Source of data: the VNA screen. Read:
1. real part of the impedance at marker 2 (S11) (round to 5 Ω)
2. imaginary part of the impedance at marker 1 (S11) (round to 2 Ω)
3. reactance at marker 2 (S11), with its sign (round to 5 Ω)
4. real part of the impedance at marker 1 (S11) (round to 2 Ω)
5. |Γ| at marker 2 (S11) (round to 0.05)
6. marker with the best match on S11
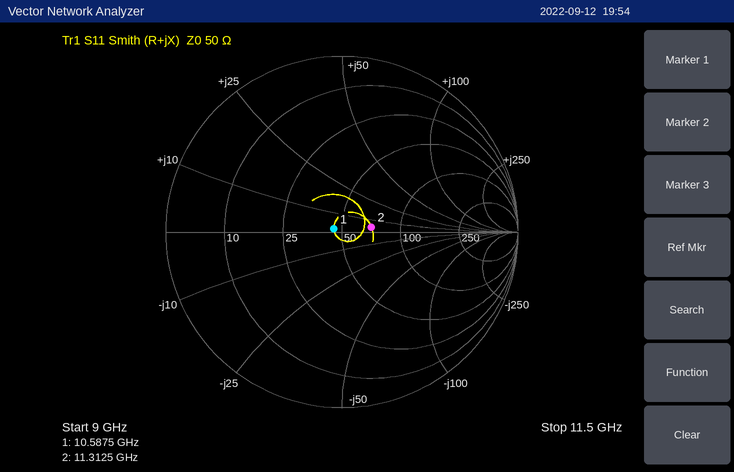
70 Ω
+2 Ω
+5 Ω
46 Ω
0.15
marker 1
